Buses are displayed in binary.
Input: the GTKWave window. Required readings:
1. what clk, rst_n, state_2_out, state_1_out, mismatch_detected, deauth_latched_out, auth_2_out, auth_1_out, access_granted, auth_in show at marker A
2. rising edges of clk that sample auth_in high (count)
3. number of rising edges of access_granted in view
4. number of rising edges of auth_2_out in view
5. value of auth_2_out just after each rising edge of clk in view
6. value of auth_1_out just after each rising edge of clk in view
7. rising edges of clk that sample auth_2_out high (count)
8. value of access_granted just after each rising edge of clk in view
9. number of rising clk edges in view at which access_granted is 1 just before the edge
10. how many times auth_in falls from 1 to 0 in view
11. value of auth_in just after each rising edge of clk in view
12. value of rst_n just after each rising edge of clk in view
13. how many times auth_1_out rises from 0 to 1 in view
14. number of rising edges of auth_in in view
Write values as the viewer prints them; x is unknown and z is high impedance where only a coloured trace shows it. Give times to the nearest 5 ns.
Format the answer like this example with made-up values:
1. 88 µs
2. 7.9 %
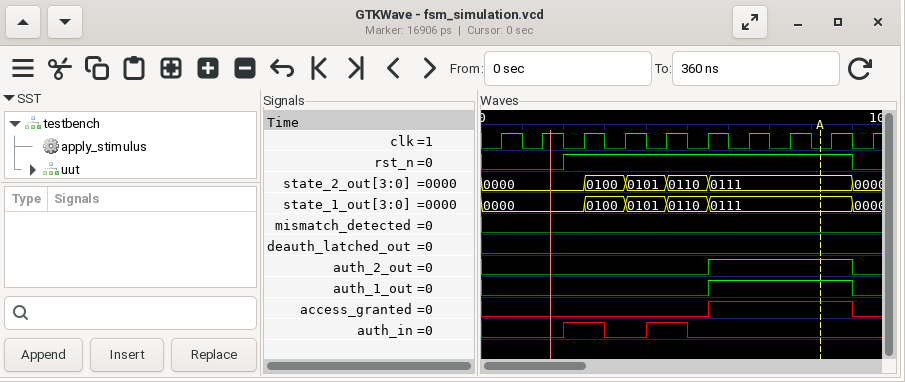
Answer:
1. clk=0, rst_n=1, state_2_out=0111, state_1_out=0111, mismatch_detected=0, deauth_latched_out=0, auth_2_out=1, auth_1_out=1, access_granted=1, auth_in=0
2. 2
3. 1
4. 1
5. 0 0 0 0 0 1 1 1 1 0
6. 0 0 0 0 0 1 1 1 1 0
7. 3
8. 0 0 0 0 0 1 1 1 1 0
9. 3
10. 2
11. 0 0 1 0 1 0 0 0 0 0
12. 0 0 1 1 1 1 1 1 1 0
13. 1
14. 2
